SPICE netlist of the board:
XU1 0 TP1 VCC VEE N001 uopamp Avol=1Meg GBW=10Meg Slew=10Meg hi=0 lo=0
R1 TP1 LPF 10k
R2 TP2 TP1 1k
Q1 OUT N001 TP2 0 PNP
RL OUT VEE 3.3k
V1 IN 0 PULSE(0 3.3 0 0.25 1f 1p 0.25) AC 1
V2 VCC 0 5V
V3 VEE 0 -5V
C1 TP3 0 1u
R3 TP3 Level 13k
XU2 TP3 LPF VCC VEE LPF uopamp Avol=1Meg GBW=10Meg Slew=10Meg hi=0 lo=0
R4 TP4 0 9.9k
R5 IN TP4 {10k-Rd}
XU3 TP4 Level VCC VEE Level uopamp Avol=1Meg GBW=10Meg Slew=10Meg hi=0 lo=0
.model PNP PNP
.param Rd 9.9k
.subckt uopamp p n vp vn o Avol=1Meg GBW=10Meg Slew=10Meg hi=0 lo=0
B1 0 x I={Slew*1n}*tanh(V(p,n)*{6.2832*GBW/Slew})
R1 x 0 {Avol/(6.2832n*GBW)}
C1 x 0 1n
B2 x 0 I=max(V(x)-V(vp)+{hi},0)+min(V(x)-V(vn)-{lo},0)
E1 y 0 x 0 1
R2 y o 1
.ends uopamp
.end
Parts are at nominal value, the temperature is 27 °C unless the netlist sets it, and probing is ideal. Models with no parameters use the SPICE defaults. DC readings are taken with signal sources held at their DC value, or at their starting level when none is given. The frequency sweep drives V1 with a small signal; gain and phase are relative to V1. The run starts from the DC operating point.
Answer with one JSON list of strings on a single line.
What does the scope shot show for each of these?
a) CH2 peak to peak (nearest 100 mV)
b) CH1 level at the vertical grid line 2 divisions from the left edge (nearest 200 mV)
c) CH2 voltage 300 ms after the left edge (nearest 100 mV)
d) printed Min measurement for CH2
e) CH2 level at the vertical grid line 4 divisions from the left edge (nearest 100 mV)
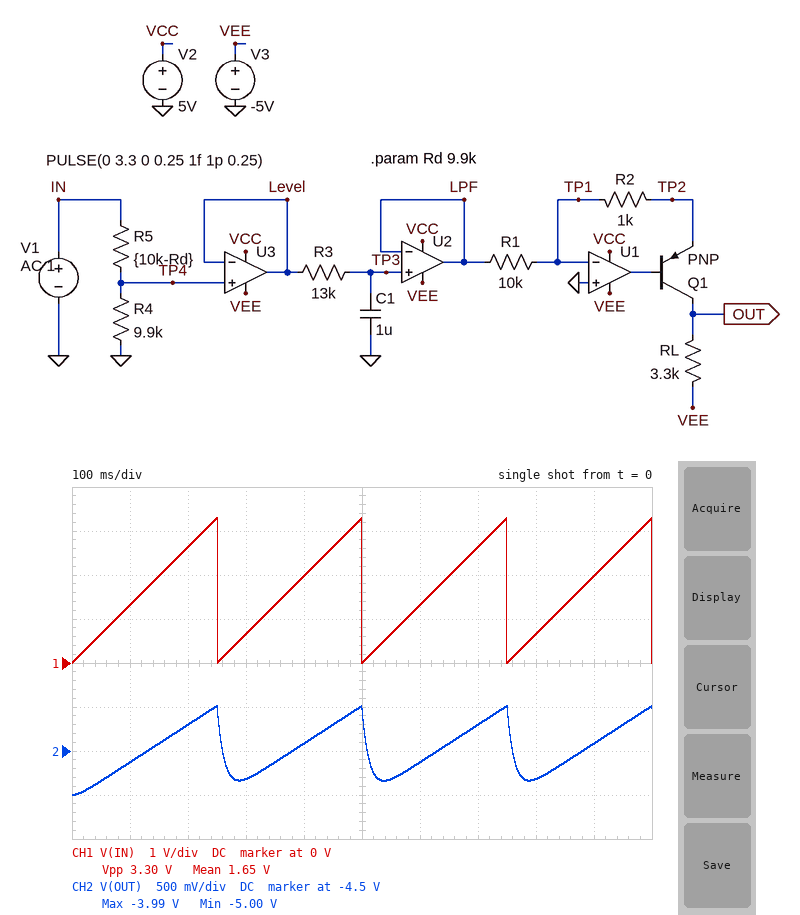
["1.0 V", "2.6 V", "-4.8 V", "-5.00 V", "-4.4 V"]
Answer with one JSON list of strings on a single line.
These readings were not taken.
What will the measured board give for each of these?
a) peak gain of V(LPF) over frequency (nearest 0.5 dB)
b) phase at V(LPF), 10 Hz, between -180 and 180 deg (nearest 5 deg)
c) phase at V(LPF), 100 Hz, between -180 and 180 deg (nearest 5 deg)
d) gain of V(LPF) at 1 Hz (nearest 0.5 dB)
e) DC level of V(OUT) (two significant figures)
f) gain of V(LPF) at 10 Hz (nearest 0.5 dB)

["0 dB", "-40 deg", "-85 deg", "0 dB", "-5.0 V", "-2.5 dB"]
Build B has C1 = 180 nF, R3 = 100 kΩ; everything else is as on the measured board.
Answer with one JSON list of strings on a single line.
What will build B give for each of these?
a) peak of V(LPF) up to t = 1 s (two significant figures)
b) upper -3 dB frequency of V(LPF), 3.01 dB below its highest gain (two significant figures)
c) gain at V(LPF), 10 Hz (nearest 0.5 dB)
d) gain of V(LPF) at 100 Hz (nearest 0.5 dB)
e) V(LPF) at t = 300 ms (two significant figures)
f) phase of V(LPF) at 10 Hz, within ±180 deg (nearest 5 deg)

["3.0 V", "8.8 Hz", "-3.5 dB", "-21.0 dB", "620 mV", "-50 deg"]
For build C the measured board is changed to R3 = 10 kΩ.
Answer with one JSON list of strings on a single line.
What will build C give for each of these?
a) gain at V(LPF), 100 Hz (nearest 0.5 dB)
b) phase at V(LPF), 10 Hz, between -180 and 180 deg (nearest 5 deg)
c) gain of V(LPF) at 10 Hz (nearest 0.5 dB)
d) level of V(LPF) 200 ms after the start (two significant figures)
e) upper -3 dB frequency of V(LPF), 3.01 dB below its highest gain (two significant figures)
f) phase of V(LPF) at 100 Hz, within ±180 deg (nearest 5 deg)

["-16.0 dB", "-30 deg", "-1.5 dB", "2.5 V", "16 Hz", "-80 deg"]
